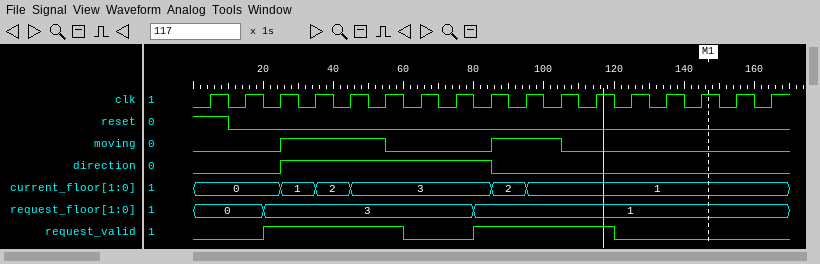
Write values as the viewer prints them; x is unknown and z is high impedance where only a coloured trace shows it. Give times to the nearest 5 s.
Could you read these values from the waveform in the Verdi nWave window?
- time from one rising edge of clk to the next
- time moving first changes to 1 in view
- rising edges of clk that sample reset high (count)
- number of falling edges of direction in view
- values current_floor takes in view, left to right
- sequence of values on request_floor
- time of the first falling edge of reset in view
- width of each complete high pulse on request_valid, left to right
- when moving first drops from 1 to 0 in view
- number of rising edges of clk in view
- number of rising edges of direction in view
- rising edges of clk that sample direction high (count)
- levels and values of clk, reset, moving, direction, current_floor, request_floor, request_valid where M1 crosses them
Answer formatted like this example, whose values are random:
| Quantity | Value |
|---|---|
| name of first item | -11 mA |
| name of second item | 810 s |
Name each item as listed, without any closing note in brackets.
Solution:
| Quantity | Value |
|---|---|
| time from one rising edge of clk to the next | 10 s |
| time moving first changes to 1 in view | 25 s |
| rising edges of clk that sample reset high | 1 |
| number of falling edges of direction in view | 1 |
| values current_floor takes in view, left to right | 0, 1, 2, 3, 2, 1 |
| sequence of values on request_floor | 0, 3, 1 |
| time of the first falling edge of reset in view | 10 s |
| width of each complete high pulse on request_valid, left to right | 40 s, 40 s |
| when moving first drops from 1 to 0 in view | 55 s |
| number of rising edges of clk in view | 17 |
| number of rising edges of direction in view | 1 |
| rising edges of clk that sample direction high | 6 |
| levels and values of clk, reset, moving, direction, current_floor, request_floor, request_valid where M1 crosses them | clk=1, reset=0, moving=0, direction=0, current_floor=1, request_floor=1, request_valid=0 |
